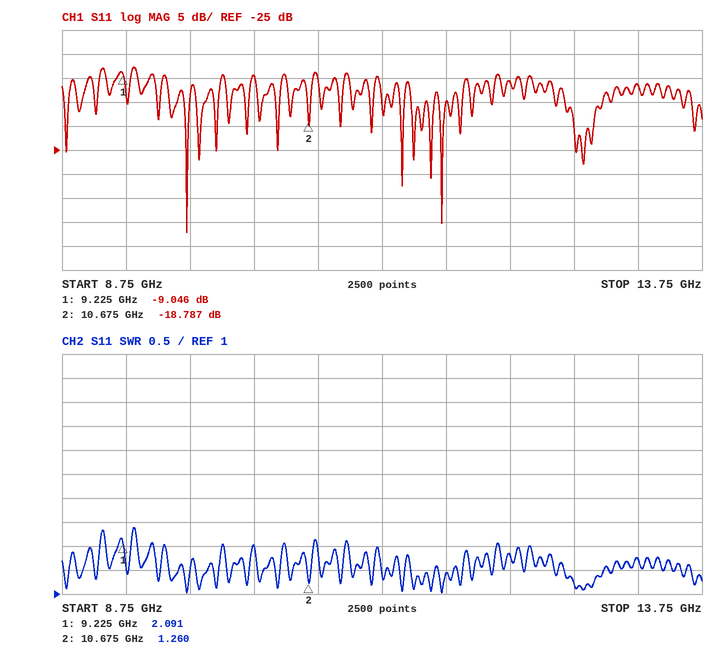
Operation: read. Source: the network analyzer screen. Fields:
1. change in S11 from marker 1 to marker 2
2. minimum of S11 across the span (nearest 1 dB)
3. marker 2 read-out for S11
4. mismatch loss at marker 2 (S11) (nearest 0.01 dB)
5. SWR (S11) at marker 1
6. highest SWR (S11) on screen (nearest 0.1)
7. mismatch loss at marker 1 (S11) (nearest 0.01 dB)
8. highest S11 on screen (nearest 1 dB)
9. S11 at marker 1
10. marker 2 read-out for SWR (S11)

-9.741 dB
-42 dB
-18.787 dB
0.06 dB
2.091
2.4
0.58 dB
-8 dB
-9.046 dB
1.260
